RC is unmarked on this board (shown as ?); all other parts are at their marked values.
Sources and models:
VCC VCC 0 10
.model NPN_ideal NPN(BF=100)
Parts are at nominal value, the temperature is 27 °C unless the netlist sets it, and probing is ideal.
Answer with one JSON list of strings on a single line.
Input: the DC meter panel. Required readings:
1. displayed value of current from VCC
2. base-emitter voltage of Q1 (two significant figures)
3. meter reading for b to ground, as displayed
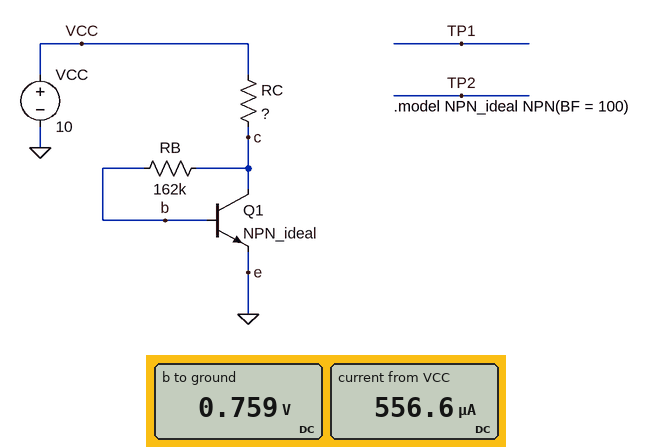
["556.6 µA", "760 mV", "0.759 V"]
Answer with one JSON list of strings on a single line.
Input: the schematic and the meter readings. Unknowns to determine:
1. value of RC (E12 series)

["15 kΩ"]
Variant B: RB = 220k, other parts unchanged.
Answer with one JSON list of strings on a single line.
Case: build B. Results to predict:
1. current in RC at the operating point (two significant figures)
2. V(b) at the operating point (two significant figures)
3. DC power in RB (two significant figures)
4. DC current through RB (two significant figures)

["540 µA", "760 mV", "6.2 µW", "5.3 µA"]
